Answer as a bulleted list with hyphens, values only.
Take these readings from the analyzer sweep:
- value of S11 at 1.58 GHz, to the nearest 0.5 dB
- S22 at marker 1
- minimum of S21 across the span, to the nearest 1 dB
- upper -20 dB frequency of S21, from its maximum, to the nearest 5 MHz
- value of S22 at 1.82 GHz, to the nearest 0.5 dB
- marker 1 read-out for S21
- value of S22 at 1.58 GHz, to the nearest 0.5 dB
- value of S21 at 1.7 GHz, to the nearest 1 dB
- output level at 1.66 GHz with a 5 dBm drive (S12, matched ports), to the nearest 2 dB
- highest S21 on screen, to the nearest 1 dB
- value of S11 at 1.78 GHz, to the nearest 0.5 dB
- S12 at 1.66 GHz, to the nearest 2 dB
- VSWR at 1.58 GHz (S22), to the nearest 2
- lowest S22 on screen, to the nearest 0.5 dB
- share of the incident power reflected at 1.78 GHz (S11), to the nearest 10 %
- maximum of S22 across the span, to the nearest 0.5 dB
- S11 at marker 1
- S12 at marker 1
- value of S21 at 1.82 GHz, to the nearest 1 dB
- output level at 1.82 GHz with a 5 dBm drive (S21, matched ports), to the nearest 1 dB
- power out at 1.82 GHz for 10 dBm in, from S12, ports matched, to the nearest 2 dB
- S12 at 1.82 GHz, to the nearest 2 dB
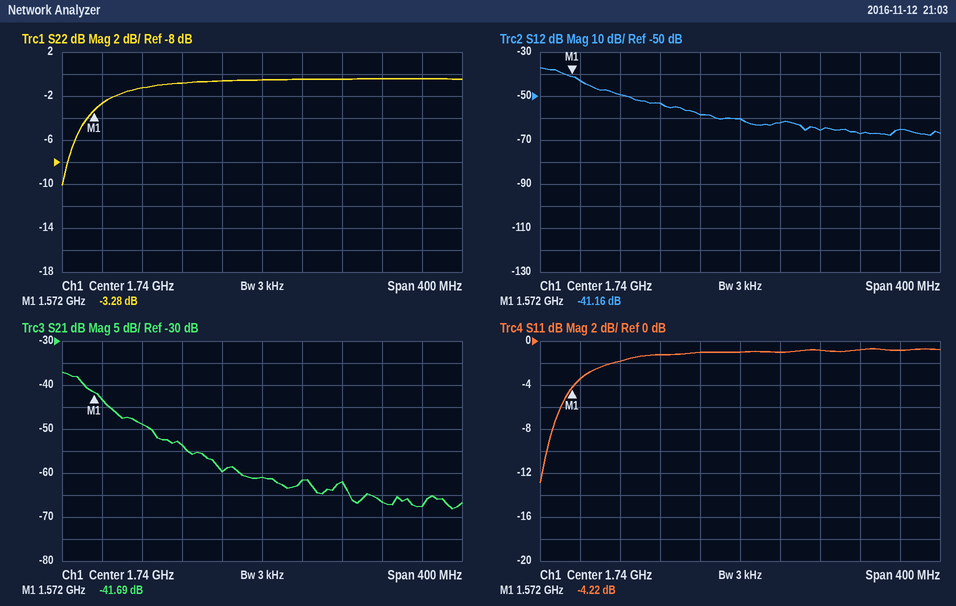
- -3.5 dB
- -3.28 dB
- -68 dB
- 1.690 GHz
- -0.5 dB
- -41.69 dB
- -2.5 dB
- -60 dB
- -48 dBm
- -37 dB
- -1.0 dB
- -54 dB
- 6
- -10.0 dB
- 80 %
- -0.5 dB
- -4.22 dB
- -41.16 dB
- -62 dB
- -57 dBm
- -56 dBm
- -66 dB
